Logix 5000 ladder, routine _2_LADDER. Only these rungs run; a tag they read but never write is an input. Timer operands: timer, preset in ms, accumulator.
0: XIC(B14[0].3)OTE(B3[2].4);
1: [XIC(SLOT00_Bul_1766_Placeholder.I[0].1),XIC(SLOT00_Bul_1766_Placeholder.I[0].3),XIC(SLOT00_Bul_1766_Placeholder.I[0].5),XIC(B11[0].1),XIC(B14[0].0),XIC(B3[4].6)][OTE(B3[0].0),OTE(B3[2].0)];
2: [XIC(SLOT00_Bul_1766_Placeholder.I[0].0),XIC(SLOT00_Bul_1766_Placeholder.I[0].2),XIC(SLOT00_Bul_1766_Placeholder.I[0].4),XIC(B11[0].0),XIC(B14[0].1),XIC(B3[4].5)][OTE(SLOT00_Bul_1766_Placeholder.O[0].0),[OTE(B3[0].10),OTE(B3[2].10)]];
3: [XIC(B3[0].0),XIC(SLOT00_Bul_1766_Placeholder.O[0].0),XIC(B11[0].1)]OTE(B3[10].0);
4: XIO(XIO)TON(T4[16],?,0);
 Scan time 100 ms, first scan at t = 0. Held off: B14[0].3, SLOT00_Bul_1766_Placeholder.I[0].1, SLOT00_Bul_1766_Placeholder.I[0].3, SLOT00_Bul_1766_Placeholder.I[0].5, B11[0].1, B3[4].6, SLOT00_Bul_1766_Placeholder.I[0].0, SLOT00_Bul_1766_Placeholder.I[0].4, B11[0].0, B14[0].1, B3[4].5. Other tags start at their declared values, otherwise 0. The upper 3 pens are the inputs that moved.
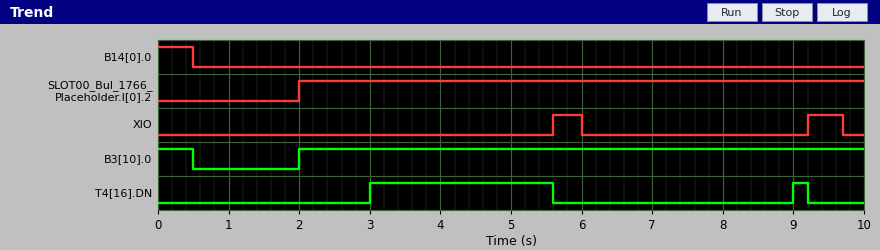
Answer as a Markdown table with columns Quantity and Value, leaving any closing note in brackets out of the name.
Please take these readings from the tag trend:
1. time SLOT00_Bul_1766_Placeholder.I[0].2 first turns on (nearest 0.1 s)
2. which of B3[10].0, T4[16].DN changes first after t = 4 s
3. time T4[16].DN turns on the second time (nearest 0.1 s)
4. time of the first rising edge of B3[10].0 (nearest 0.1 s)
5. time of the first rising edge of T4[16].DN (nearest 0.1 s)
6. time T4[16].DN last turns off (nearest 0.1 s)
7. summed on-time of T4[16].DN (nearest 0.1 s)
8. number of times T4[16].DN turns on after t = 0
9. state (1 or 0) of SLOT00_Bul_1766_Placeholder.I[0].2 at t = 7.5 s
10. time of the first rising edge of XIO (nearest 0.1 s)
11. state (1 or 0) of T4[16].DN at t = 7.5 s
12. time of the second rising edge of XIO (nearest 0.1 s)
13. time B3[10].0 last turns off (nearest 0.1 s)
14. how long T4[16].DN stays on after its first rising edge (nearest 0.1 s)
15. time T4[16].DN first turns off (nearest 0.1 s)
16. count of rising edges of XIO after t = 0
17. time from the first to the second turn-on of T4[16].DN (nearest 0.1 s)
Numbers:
| Quantity | Value |
|---|---|
| time SLOT00_Bul_1766_Placeholder.I[0].2 first turns on | 2.0 s |
| which of B3[10].0, T4[16].DN changes first after t = 4 s | T4[16].DN |
| time T4[16].DN turns on the second time | 9.0 s |
| time of the first rising edge of B3[10].0 | 2.0 s |
| time of the first rising edge of T4[16].DN | 3.0 s |
| time T4[16].DN last turns off | 9.2 s |
| summed on-time of T4[16].DN | 2.8 s |
| number of times T4[16].DN turns on after t = 0 | 2 |
| state (1 or 0) of SLOT00_Bul_1766_Placeholder.I[0].2 at t = 7.5 s | 1 |
| time of the first rising edge of XIO | 5.6 s |
| state (1 or 0) of T4[16].DN at t = 7.5 s | 0 |
| time of the second rising edge of XIO | 9.2 s |
| time B3[10].0 last turns off | 0.5 s |
| how long T4[16].DN stays on after its first rising edge | 2.6 s |
| time T4[16].DN first turns off | 5.6 s |
| count of rising edges of XIO after t = 0 | 2 |
| time from the first to the second turn-on of T4[16].DN | 6.0 s |
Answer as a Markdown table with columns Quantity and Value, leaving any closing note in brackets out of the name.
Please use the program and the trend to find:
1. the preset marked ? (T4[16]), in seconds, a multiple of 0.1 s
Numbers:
| Quantity | Value |
|---|---|
| the preset marked ? (T4[16]), in seconds, a multiple of 0.1 s | 3.0 s |
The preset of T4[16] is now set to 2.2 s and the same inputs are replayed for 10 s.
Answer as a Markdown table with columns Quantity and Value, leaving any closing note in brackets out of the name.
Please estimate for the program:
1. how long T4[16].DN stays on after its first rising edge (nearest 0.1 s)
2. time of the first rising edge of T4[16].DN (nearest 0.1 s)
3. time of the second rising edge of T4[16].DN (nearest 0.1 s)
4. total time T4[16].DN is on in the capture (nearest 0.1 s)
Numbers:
| Quantity | Value |
|---|---|
| how long T4[16].DN stays on after its first rising edge | 3.4 s |
| time of the first rising edge of T4[16].DN | 2.2 s |
| time of the second rising edge of T4[16].DN | 8.2 s |
| total time T4[16].DN is on in the capture | 4.4 s |
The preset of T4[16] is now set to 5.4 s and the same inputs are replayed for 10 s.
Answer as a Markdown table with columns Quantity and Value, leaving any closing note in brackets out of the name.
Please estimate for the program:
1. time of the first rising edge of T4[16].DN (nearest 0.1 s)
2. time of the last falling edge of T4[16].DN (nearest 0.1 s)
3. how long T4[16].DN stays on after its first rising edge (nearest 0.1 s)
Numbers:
| Quantity | Value |
|---|---|
| time of the first rising edge of T4[16].DN | 5.4 s |
| time of the last falling edge of T4[16].DN | 5.6 s |
| how long T4[16].DN stays on after its first rising edge | 0.2 s |
